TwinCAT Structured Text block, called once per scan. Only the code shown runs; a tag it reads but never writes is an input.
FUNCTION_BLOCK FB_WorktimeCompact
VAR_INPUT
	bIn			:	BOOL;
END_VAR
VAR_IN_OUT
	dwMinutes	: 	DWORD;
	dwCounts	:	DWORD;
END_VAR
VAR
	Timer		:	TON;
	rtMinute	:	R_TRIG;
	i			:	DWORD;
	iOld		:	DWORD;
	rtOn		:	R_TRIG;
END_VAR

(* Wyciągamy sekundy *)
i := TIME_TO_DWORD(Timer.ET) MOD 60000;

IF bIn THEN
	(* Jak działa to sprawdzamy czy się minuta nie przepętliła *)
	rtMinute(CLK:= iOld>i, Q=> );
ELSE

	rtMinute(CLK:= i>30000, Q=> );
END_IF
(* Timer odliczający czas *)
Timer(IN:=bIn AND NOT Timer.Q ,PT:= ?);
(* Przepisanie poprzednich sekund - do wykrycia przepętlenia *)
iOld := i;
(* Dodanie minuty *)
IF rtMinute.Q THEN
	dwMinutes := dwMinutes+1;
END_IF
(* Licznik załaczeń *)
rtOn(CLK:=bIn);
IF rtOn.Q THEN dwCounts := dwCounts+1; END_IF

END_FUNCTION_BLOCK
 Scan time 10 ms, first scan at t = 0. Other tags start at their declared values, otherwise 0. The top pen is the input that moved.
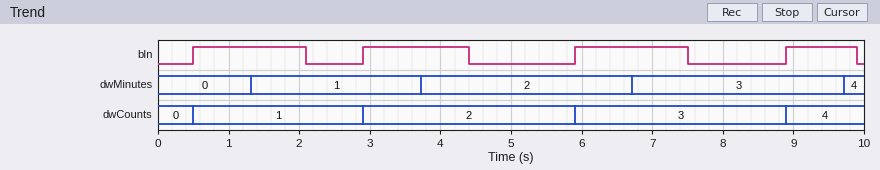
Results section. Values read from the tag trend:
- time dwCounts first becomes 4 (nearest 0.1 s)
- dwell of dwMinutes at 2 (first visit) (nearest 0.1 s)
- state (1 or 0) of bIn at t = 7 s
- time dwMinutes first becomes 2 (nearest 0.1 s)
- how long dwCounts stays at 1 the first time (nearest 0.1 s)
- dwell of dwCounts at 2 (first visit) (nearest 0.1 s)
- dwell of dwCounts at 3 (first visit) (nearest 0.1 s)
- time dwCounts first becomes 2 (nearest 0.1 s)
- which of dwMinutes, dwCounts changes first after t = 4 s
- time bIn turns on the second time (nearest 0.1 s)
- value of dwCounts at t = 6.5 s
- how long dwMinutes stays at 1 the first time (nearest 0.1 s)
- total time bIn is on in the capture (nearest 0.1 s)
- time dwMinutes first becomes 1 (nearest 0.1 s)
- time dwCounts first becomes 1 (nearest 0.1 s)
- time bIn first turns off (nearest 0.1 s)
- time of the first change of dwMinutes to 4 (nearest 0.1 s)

8.9 s
3.0 s
1
3.7 s
2.4 s
3.0 s
3.0 s
2.9 s
dwCounts
2.9 s
3
2.4 s
5.7 s
1.3 s
0.5 s
2.1 s
9.7 s
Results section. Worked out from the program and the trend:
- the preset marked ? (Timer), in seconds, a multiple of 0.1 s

0.8 s
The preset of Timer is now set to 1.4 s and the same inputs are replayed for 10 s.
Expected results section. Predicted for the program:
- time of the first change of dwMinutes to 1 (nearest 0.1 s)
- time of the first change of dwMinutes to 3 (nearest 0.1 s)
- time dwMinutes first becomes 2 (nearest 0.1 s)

1.9 s
7.3 s
4.3 s
